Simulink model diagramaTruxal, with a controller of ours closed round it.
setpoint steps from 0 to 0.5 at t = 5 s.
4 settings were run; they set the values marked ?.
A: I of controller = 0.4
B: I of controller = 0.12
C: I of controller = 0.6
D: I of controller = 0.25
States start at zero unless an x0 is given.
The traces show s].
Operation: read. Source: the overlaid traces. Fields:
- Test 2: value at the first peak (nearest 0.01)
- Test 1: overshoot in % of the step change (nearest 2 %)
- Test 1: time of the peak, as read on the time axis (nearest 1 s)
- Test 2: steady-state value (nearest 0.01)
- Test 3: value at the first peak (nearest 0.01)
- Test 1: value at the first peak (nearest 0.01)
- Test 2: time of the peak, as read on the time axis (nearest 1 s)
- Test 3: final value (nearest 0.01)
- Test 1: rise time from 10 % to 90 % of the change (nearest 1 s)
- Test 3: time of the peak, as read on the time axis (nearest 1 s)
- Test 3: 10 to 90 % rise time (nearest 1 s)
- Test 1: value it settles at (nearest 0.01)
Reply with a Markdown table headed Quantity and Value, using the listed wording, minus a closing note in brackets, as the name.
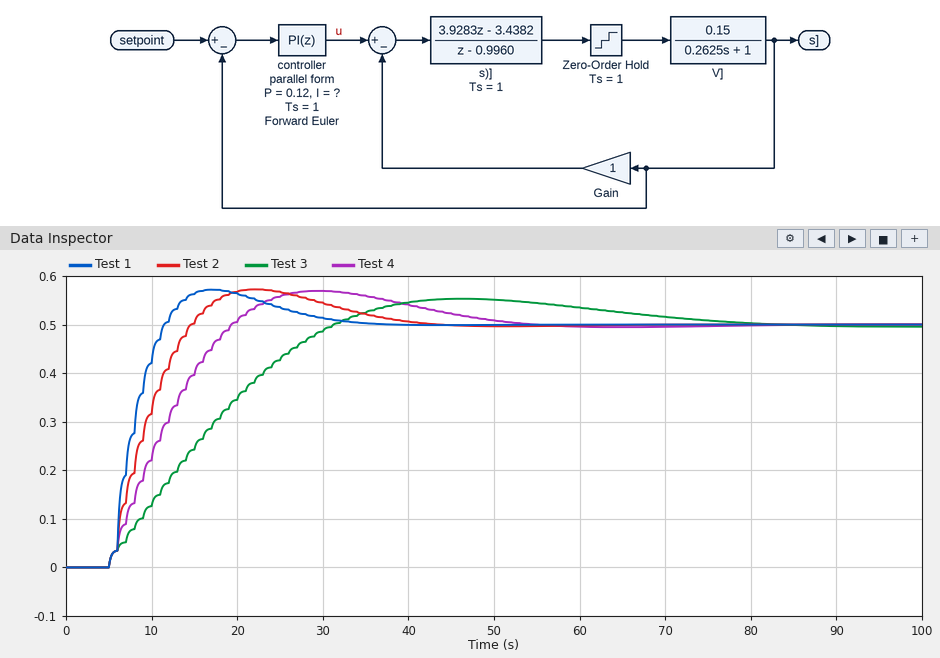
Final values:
| Quantity | Value |
|---|---|
| Test 2: value at the first peak | 0.57 |
| Test 1: overshoot in % of the step change | 14 % |
| Test 1: time of the peak, as read on the time axis | 17 s |
| Test 2: steady-state value | 0.50 |
| Test 3: value at the first peak | 0.55 |
| Test 1: value at the first peak | 0.57 |
| Test 2: time of the peak, as read on the time axis | 22 s |
| Test 3: final value | 0.50 |
| Test 1: rise time from 10 % to 90 % of the change | 4 s |
| Test 3: time of the peak, as read on the time axis | 47 s |
| Test 3: 10 to 90 % rise time | 20 s |
| Test 1: value it settles at | 0.50 |
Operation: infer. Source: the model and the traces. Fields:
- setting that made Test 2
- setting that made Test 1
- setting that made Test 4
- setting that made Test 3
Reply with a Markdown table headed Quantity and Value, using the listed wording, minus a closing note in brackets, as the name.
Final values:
| Quantity | Value |
|---|---|
| setting that made Test 2 | A |
| setting that made Test 1 | C |
| setting that made Test 4 | D |
| setting that made Test 3 | B |
